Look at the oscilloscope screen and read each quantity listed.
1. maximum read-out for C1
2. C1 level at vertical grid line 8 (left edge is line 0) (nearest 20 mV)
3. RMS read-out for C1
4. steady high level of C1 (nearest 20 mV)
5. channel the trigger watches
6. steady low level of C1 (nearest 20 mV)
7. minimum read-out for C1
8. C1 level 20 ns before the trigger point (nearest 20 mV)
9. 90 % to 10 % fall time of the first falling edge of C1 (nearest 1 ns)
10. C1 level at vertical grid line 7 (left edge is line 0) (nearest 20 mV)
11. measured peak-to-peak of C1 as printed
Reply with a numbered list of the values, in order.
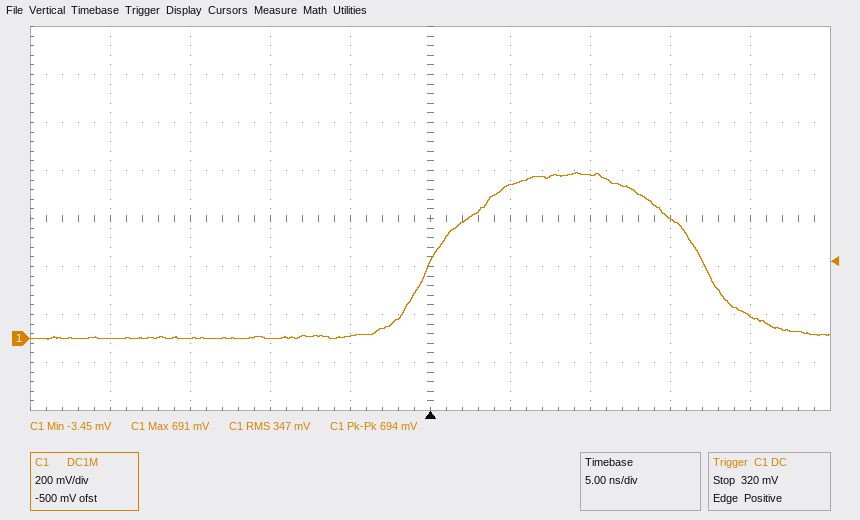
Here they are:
1. 691 mV
2. 500 mV
3. 347 mV
4. 680 mV
5. C1
6. 0 mV
7. -3.45 mV
8. 0 mV
9. 8 ns
10. 680 mV
11. 694 mV
